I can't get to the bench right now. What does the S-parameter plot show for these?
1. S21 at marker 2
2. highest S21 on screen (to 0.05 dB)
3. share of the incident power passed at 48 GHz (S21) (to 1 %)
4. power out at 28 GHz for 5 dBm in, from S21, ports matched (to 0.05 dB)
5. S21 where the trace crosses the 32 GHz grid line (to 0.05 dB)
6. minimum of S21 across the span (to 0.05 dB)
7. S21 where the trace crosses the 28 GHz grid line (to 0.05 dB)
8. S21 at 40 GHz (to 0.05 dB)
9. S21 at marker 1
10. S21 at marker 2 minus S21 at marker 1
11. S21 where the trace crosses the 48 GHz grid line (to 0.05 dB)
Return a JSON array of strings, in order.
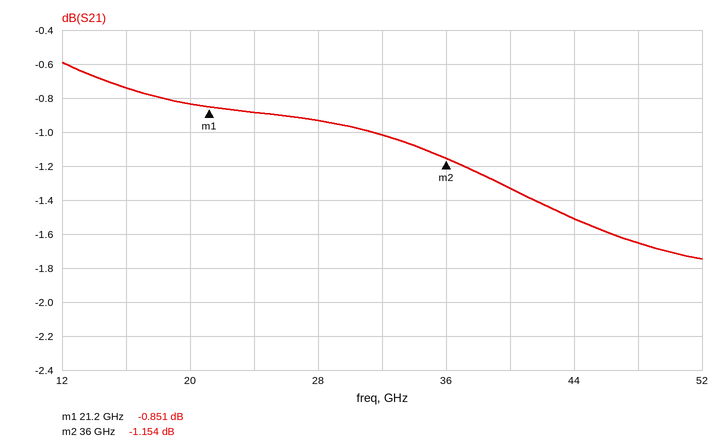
["-1.154 dB", "-0.60 dB", "68 %", "4.05 dBm", "-1.00 dB", "-1.75 dB", "-0.95 dB", "-1.35 dB", "-0.851 dB", "-0.303 dB", "-1.65 dB"]
